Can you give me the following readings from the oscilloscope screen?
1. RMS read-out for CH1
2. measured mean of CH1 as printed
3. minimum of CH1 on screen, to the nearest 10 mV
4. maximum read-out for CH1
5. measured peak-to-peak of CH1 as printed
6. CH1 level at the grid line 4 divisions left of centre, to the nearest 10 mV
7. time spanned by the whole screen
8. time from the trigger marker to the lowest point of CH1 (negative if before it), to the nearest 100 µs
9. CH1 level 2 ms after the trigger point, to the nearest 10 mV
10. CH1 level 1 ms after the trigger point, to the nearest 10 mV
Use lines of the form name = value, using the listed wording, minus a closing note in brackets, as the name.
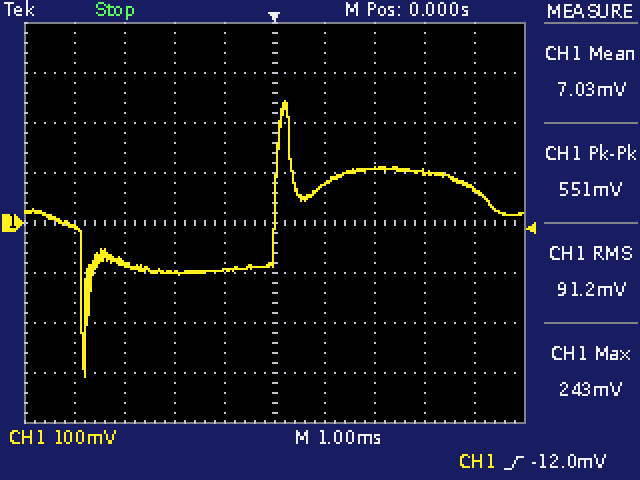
RMS read-out for CH1 = 91.2 mV
measured mean of CH1 as printed = 7.03 mV
minimum of CH1 on screen, to the nearest 10 mV = -310 mV
maximum read-out for CH1 = 243 mV
measured peak-to-peak of CH1 as printed = 551 mV
CH1 level at the grid line 4 divisions left of centre, to the nearest 10 mV = -10 mV
time spanned by the whole screen = 10 ms
time from the trigger marker to the lowest point of CH1 (negative if before it), to the nearest 100 µs = -3.8 ms
CH1 level 2 ms after the trigger point, to the nearest 10 mV = 110 mV
CH1 level 1 ms after the trigger point, to the nearest 10 mV = 80 mV
